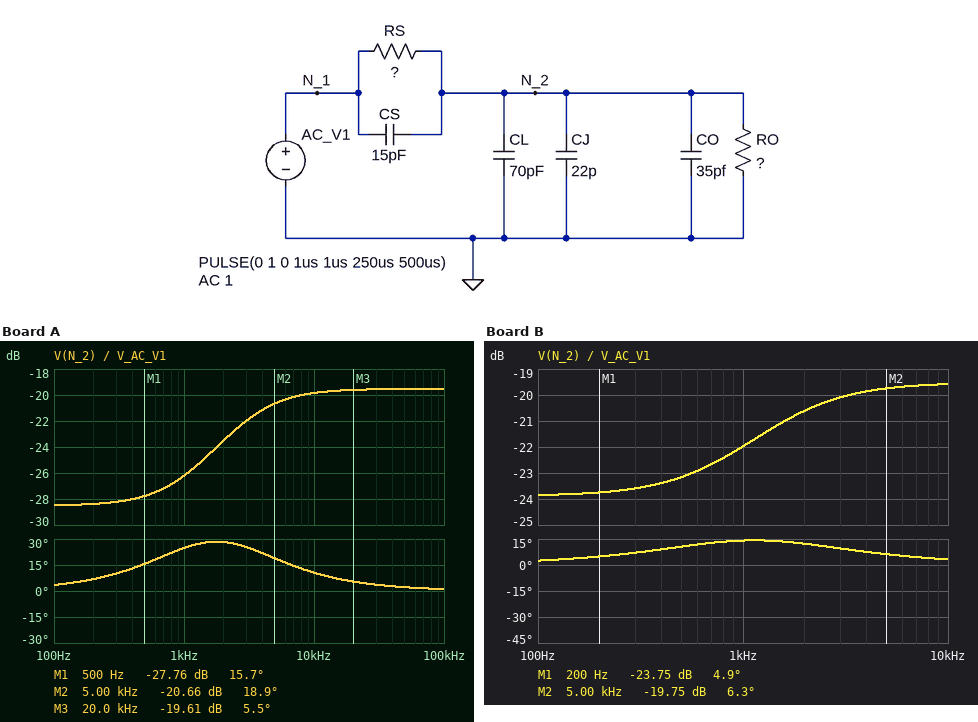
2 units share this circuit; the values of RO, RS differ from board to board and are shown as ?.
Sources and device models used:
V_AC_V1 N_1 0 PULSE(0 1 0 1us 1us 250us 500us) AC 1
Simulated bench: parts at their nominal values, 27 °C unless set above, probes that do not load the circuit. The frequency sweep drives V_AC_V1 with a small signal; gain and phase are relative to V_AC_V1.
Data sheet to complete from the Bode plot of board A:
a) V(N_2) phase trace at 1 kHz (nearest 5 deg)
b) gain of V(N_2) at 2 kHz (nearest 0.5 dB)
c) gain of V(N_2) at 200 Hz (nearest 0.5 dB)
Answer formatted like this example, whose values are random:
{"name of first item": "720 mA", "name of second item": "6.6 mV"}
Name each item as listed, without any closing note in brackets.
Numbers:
{"V(N_2) phase trace at 1 kHz": "25 deg", "gain of V(N_2) at 2 kHz": "-23.5 dB", "gain of V(N_2) at 200 Hz": "-28.5 dB"}
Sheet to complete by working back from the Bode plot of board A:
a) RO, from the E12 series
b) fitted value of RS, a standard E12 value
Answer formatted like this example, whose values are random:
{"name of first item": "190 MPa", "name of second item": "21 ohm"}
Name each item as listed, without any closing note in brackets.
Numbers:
{"RO, from the E12 series": "390 kΩ", "fitted value of RS, a standard E12 value": "10 MΩ"}
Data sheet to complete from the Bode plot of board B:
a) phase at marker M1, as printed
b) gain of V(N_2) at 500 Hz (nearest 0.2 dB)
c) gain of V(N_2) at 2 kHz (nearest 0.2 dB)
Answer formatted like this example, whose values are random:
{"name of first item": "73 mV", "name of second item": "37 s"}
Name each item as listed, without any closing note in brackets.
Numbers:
{"phase at marker M1, as printed": "4.9 deg", "gain of V(N_2) at 500 Hz": "-23.2 dB", "gain of V(N_2) at 2 kHz": "-20.6 dB"}
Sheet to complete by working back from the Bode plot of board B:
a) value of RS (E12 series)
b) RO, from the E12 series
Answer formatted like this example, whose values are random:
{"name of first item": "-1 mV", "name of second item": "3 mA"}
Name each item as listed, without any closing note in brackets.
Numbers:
{"value of RS": "12 MΩ", "RO, from the E12 series": "820 kΩ"}
